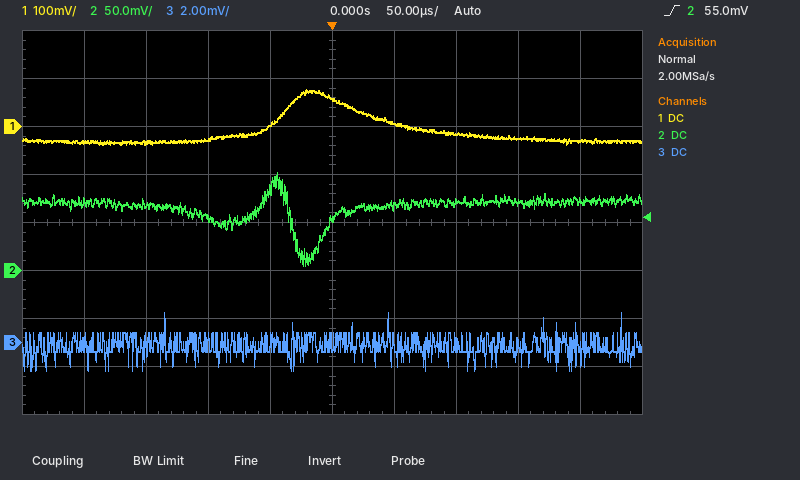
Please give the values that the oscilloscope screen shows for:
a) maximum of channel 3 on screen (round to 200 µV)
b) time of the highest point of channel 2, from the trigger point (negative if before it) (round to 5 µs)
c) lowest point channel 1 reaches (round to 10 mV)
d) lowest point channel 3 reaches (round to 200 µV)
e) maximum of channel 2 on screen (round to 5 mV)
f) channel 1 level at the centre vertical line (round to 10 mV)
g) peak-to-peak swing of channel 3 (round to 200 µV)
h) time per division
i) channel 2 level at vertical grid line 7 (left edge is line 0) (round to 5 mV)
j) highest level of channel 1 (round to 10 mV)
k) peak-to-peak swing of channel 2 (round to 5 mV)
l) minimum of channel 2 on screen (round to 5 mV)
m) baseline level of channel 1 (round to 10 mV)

1.2 mV
-45 µs
-40 mV
-1.2 mV
100 mV
60 mV
2.4 mV
50 µs
70 mV
80 mV
95 mV
5 mV
-30 mV
